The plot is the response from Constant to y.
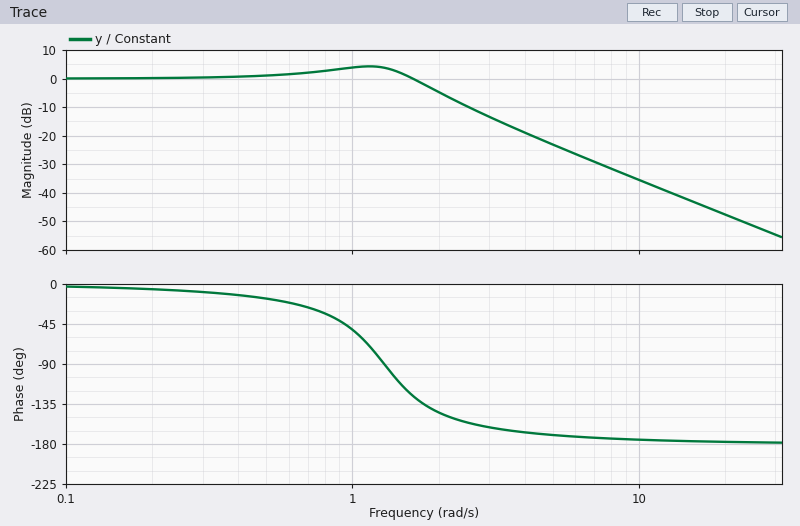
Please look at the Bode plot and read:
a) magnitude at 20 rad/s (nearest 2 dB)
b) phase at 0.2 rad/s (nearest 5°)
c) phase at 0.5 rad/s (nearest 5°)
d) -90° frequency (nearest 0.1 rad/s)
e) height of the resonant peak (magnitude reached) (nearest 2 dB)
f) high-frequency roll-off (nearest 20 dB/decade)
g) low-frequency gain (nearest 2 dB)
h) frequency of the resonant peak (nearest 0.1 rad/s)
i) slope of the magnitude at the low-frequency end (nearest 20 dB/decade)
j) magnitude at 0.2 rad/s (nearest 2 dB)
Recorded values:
-48 dB
-5°
-15°
1.3 rad/s
4 dB
-40 dB/decade
0 dB
1.1 rad/s
0 dB/decade
0 dB
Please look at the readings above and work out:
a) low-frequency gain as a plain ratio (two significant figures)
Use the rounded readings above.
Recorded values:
1.0
